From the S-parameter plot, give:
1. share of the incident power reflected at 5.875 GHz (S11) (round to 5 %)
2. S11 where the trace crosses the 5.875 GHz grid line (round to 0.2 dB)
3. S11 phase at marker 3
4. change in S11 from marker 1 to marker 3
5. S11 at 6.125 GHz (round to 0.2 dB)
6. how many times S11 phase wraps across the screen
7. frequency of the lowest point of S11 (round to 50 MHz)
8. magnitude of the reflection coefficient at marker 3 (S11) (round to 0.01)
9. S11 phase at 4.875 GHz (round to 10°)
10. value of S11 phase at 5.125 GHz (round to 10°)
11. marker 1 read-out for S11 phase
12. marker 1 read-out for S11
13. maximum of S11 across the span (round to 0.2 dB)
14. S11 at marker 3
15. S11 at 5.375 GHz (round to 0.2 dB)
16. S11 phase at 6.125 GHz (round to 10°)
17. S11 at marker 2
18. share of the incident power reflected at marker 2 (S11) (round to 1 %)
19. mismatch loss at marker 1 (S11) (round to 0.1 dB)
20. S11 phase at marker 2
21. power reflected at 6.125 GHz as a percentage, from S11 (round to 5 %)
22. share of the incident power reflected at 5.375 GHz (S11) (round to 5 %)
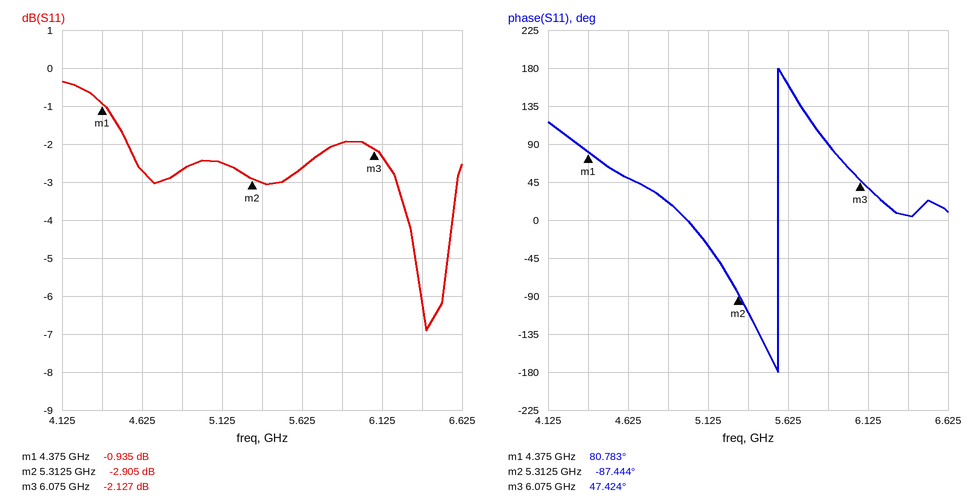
65 %
-2.0 dB
47.424°
-1.192 dB
-2.4 dB
1
6.40 GHz
0.78
20°
-30°
80.783°
-0.935 dB
-0.4 dB
-2.127 dB
-3.0 dB
40°
-2.905 dB
51 %
7.1 dB
-87.444°
60 %
50 %
